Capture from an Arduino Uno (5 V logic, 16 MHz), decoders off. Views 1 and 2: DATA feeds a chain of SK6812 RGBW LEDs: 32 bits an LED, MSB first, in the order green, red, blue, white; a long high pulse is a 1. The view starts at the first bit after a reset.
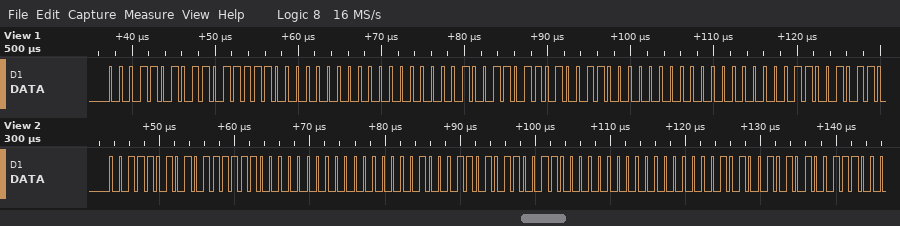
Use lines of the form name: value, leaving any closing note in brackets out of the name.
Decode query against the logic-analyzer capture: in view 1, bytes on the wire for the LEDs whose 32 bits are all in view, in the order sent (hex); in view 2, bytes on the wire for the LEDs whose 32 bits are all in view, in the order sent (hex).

in view 1, bytes on the wire for the LEDs whose 32 bits are all in view, in the order sent: 1A DF 00 00 26 D3 00 00
in view 2, bytes on the wire for the LEDs whose 32 bits are all in view, in the order sent: 3A BF 00 00 46 B3 00 00
